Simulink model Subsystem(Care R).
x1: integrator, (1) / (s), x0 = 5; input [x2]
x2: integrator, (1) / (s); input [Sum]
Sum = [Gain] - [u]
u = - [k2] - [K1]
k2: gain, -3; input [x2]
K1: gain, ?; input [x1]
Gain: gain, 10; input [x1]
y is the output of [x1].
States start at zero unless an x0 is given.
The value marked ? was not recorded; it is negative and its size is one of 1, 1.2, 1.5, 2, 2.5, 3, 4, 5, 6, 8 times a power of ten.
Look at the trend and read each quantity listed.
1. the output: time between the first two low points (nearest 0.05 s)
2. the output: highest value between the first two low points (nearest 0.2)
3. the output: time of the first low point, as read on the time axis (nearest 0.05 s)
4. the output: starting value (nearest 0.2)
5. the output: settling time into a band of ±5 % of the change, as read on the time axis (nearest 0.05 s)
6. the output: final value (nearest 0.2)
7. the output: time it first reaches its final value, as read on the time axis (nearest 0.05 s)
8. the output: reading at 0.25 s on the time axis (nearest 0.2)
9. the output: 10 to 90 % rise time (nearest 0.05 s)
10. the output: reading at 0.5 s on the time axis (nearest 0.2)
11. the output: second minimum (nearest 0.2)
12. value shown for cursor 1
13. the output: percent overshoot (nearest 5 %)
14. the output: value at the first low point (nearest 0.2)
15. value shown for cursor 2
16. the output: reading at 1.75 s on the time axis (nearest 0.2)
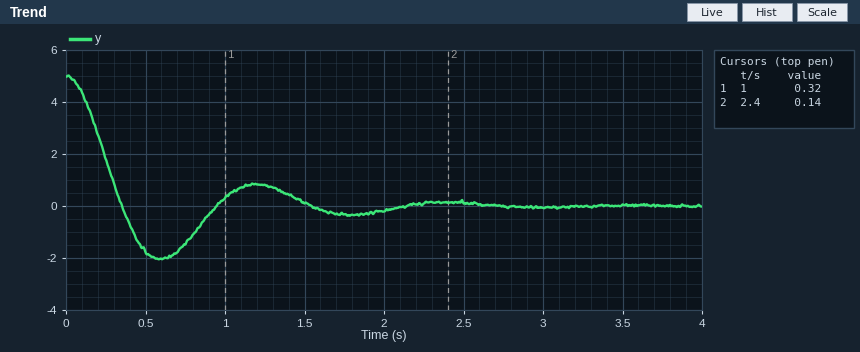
1.20 s
0.8
0.60 s
5.0
1.95 s
0.0
0.35 s
1.8
0.25 s
-1.8
-0.4
0.32
40 %
-2.0
0.14
-0.4
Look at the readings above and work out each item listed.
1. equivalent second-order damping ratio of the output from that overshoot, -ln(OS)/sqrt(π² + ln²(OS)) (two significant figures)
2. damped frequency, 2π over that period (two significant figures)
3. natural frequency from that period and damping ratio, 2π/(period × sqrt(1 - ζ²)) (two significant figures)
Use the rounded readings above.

0.28
5.2 rad/s
5.5 rad/s
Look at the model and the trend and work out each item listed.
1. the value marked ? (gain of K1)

-40
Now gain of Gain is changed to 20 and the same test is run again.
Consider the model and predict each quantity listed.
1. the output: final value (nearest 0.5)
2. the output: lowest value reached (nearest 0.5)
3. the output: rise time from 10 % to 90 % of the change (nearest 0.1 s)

0.0
-1.5
0.3 s
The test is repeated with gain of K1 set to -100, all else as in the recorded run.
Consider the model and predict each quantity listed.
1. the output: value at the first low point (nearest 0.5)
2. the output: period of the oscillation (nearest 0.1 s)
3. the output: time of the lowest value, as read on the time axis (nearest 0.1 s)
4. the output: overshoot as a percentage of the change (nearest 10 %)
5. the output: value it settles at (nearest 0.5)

-3.0
0.7 s
0.3 s
60 %
0.0
